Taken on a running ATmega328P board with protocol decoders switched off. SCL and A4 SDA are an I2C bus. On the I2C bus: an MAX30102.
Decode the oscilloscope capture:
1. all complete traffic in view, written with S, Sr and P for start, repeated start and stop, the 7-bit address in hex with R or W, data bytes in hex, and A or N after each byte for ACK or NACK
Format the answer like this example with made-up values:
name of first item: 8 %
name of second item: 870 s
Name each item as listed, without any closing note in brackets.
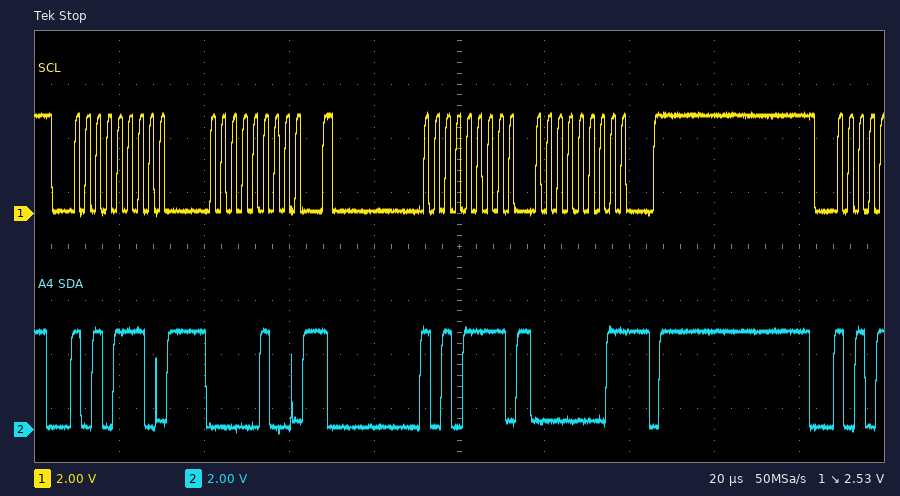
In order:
all complete traffic in view, written with S, Sr and P for start, repeated start and stop, the 7-bit address in hex with R or W, data bytes in hex, and A or N after each byte for ACK or NACK: S 57W A 04 A Sr 57R A 01 N P
